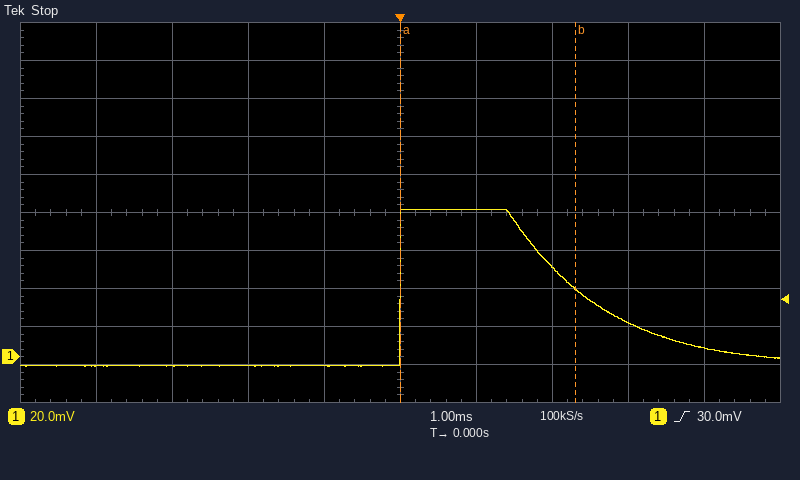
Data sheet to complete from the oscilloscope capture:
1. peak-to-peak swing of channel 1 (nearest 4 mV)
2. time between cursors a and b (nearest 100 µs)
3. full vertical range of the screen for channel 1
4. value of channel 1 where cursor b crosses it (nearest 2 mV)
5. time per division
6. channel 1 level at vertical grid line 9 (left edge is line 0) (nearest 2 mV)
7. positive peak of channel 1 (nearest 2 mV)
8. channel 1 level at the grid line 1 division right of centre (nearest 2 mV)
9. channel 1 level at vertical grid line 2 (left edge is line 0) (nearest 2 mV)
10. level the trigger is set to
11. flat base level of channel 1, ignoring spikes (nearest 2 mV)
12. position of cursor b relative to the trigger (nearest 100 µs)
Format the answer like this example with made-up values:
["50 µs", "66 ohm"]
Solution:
["84 mV", "2.3 ms", "200 mV", "36 mV", "1 ms", "4 mV", "78 mV", "78 mV", "-4 mV", "30.0 mV", "-4 mV", "+2.3 ms"]
